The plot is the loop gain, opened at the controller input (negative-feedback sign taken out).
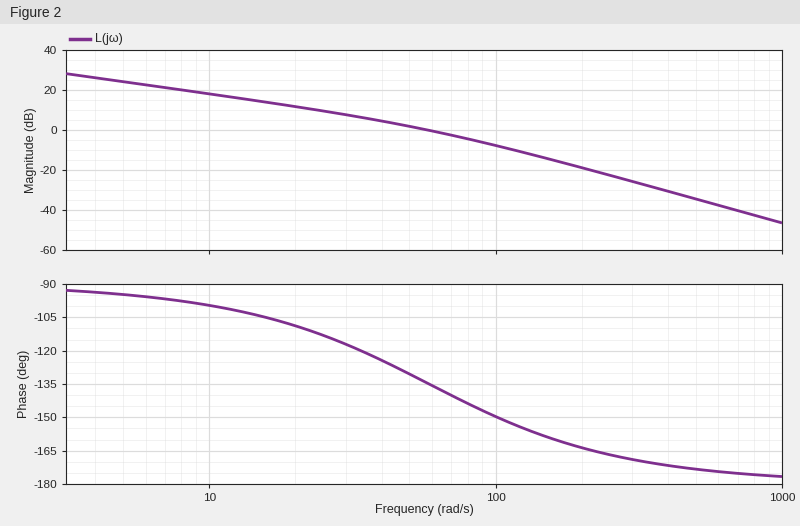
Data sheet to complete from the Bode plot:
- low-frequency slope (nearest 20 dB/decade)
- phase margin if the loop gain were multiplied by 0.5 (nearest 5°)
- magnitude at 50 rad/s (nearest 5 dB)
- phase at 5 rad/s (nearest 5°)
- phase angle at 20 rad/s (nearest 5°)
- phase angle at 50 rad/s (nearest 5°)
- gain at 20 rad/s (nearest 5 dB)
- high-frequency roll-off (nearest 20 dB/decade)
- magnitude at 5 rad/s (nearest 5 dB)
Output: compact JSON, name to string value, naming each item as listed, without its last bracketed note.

{"low-frequency slope": "-20 dB/decade", "phase margin if the loop gain were multiplied by 0.5": "60°", "magnitude at 50 rad/s": "0 dB", "phase at 5 rad/s": "-95°", "phase angle at 20 rad/s": "-110°", "phase angle at 50 rad/s": "-130°", "gain at 20 rad/s": "10 dB", "high-frequency roll-off": "-40 dB/decade", "magnitude at 5 rad/s": "25 dB"}
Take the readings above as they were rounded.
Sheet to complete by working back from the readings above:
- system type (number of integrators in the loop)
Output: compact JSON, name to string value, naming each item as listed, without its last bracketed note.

{"system type": "1"}
